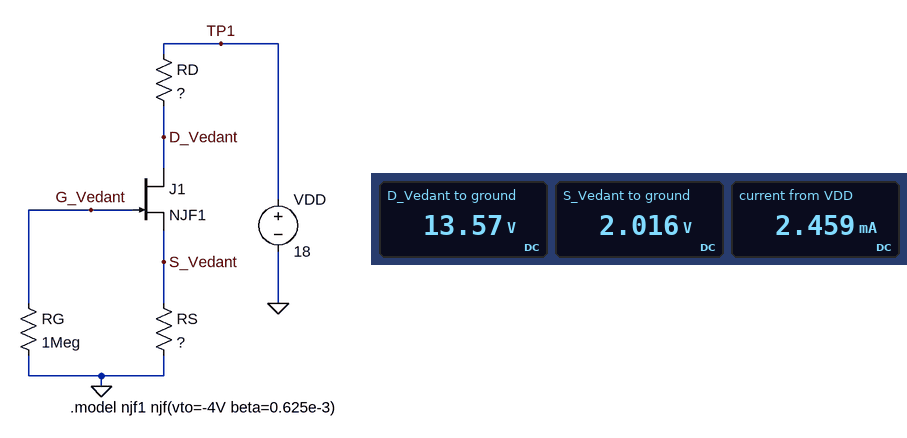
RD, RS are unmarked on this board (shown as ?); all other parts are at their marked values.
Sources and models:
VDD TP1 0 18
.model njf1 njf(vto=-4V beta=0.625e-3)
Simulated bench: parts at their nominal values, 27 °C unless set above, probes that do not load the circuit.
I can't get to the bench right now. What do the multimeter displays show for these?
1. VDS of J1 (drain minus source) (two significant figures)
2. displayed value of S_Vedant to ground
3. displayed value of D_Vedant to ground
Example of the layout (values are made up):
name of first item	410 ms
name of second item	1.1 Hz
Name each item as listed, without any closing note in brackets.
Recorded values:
VDS of J1 (drain minus source)	12 V
displayed value of S_Vedant to ground	2.016 V
displayed value of D_Vedant to ground	13.57 V
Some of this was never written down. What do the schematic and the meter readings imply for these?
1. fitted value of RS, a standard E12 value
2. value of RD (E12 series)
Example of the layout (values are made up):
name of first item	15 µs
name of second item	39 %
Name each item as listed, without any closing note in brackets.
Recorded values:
fitted value of RS, a standard E12 value	820 Ω
value of RD	1.8 kΩ
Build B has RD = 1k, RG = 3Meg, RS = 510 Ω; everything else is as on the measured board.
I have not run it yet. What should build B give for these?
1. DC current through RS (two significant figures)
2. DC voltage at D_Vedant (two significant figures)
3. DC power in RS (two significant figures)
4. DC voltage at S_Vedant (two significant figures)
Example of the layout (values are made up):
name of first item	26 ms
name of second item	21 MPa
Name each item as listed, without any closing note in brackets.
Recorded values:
DC current through RS	3.3 mA
DC voltage at D_Vedant	15 V
DC power in RS	5.6 mW
DC voltage at S_Vedant	1.7 V
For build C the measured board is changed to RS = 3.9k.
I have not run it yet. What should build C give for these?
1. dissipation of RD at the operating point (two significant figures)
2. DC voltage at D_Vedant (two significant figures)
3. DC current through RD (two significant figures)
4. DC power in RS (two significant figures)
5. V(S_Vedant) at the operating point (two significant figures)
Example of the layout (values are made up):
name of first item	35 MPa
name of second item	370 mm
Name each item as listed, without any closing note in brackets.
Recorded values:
dissipation of RD at the operating point	1.0 mW
DC voltage at D_Vedant	17 V
DC current through RD	750 µA
DC power in RS	2.2 mW
V(S_Vedant) at the operating point	2.9 V
